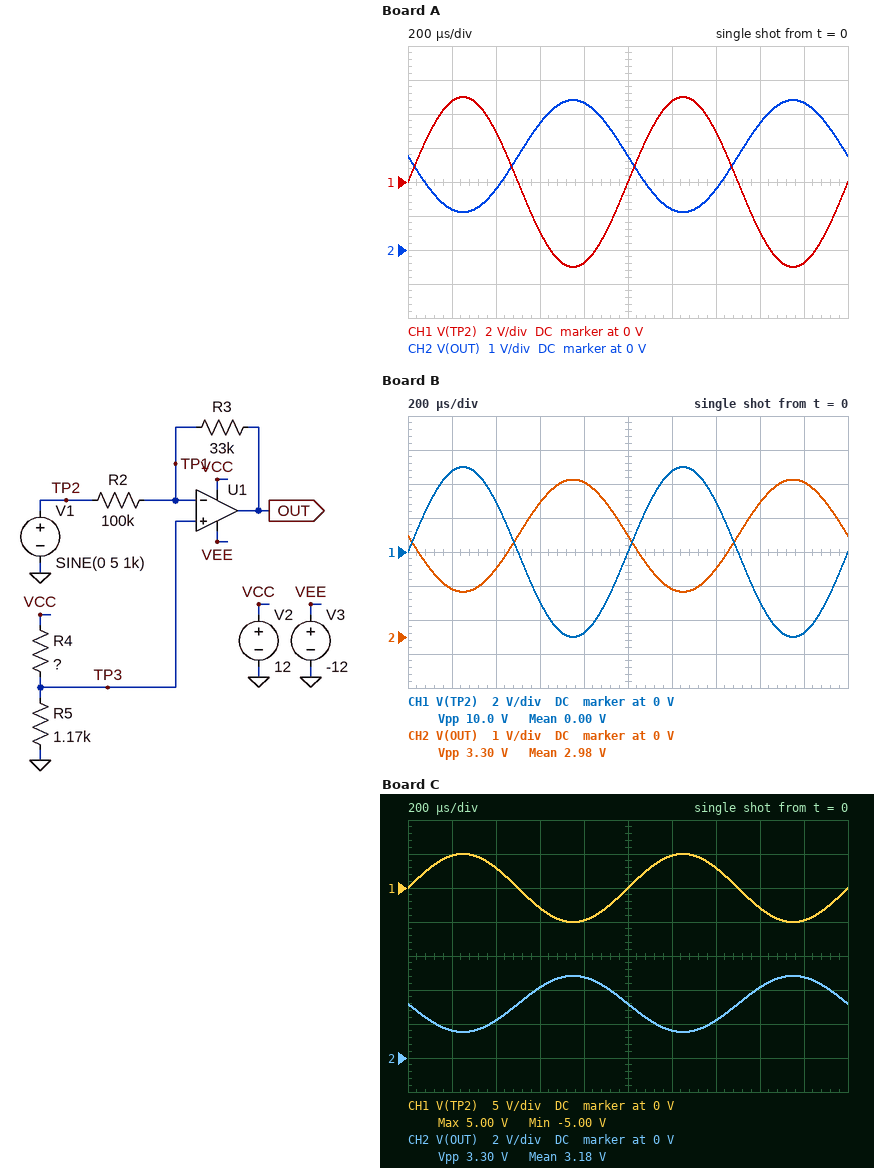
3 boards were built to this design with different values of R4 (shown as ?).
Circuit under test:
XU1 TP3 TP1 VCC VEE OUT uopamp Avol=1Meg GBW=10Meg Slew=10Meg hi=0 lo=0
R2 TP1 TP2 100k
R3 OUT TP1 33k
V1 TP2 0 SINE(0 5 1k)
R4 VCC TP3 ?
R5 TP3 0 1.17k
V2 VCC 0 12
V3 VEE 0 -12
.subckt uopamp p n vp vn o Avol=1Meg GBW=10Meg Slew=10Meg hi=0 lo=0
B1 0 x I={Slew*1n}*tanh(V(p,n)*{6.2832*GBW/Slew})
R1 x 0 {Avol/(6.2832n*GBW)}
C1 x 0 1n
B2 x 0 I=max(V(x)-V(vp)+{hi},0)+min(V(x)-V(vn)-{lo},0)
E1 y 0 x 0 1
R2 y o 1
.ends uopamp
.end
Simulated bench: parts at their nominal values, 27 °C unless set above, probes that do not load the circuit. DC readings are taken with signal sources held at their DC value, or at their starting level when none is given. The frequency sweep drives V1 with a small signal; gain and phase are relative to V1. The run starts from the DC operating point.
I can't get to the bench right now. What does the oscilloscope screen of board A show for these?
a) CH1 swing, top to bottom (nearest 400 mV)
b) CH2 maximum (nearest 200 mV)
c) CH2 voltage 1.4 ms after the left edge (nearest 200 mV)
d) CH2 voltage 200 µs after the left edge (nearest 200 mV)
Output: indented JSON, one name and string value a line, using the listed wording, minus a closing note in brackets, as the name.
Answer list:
{
  "CH1 swing, top to bottom": "10.0 V",
  "CH2 maximum": "4.4 V",
  "CH2 voltage 1.4 ms after the left edge": "1.8 V",
  "CH2 voltage 200 µs after the left edge": "1.2 V"
}
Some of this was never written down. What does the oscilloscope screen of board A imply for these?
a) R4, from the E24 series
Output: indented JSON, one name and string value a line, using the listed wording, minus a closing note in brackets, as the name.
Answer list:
{
  "R4, from the E24 series": "5.6 kΩ"
}
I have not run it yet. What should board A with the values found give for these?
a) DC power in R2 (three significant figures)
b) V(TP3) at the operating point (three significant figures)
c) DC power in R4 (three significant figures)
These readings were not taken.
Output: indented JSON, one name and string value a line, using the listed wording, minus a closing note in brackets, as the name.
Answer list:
{
  "DC power in R2": "43.0 µW",
  "V(TP3) at the operating point": "2.07 V",
  "DC power in R4": "17.6 mW"
}
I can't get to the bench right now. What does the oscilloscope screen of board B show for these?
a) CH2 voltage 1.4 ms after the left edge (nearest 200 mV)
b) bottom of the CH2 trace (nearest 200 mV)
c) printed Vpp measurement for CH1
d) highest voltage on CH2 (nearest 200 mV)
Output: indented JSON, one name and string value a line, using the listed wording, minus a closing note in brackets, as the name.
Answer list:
{
  "CH2 voltage 1.4 ms after the left edge": "2.0 V",
  "bottom of the CH2 trace": "1.4 V",
  "printed Vpp measurement for CH1": "10.0 V",
  "highest voltage on CH2": "4.6 V"
}
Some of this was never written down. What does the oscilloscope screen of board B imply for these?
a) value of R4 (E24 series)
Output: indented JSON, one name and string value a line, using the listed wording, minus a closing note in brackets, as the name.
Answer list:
{
  "value of R4": "5.1 kΩ"
}
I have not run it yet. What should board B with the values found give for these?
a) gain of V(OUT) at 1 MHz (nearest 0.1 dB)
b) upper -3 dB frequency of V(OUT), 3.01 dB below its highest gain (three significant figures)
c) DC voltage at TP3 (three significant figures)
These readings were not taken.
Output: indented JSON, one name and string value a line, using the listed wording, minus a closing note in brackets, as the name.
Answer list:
{
  "gain of V(OUT) at 1 MHz": "-9.7 dB",
  "upper -3 dB frequency of V(OUT), 3.01 dB below its highest gain": "7.52 MHz",
  "DC voltage at TP3": "2.24 V"
}
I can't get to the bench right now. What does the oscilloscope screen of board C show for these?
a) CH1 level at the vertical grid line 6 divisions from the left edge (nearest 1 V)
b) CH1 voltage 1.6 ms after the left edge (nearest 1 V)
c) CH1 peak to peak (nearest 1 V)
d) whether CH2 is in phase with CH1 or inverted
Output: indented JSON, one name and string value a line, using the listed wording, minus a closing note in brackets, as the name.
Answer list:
{
  "CH1 level at the vertical grid line 6 divisions from the left edge": "5 V",
  "CH1 voltage 1.6 ms after the left edge": "-3 V",
  "CH1 peak to peak": "10 V",
  "whether CH2 is in phase with CH1 or inverted": "inverted"
}
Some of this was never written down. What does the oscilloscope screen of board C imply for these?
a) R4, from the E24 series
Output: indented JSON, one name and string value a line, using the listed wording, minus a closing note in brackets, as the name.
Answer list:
{
  "R4, from the E24 series": "4.7 kΩ"
}
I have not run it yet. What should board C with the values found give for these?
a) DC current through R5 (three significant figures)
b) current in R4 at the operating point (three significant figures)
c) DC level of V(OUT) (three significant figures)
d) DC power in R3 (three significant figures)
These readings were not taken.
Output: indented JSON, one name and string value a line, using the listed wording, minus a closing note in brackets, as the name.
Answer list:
{
  "DC current through R5": "2.04 mA",
  "current in R4 at the operating point": "2.04 mA",
  "DC level of V(OUT)": "3.18 V",
  "DC power in R3": "18.9 µW"
}
